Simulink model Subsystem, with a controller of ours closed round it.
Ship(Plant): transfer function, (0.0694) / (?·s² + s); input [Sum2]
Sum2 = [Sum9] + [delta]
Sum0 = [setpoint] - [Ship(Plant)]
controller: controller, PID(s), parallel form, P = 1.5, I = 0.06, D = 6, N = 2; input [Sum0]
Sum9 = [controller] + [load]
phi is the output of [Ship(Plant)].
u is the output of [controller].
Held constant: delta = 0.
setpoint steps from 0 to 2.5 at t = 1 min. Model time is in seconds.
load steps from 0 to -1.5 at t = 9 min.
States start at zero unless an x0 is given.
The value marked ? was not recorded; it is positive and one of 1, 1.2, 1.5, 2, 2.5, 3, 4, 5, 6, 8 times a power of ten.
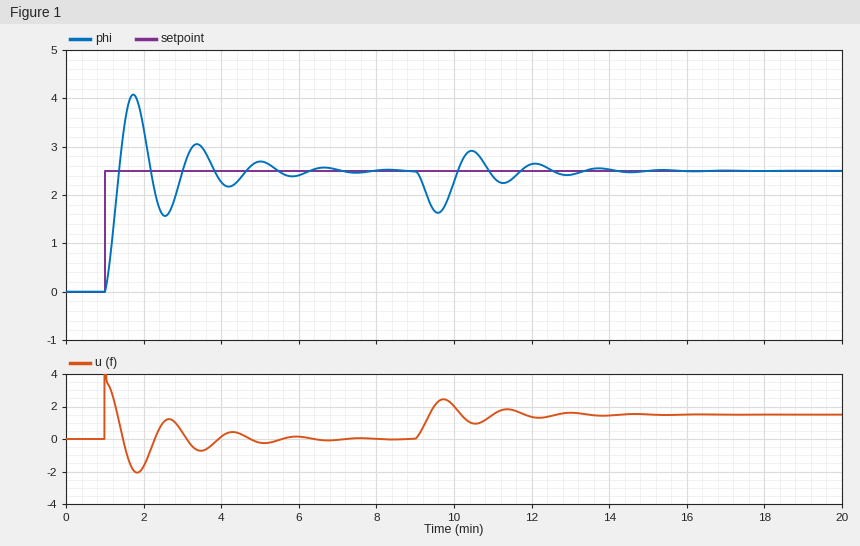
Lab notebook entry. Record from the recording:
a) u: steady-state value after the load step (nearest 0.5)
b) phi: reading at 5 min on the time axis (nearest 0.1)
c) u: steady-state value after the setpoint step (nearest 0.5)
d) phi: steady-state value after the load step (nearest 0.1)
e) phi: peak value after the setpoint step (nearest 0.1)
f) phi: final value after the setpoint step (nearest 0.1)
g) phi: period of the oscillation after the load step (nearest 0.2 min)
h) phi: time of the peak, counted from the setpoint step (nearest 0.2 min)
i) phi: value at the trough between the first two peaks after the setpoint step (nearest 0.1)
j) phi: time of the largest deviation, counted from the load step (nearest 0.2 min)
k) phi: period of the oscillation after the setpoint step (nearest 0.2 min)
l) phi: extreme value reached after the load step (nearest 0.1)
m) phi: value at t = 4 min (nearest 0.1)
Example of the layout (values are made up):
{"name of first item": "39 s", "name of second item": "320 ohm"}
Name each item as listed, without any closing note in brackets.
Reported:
{"u: steady-state value after the load step": "1.5", "phi: reading at 5 min on the time axis": "2.7", "u: steady-state value after the setpoint step": "0.0", "phi: steady-state value after the load step": "2.5", "phi: peak value after the setpoint step": "4.1", "phi: final value after the setpoint step": "2.5", "phi: period of the oscillation after the load step": "1.6 min", "phi: time of the peak, counted from the setpoint step": "0.8 min", "phi: value at the trough between the first two peaks after the setpoint step": "1.6", "phi: time of the largest deviation, counted from the load step": "0.6 min", "phi: period of the oscillation after the setpoint step": "1.6 min", "phi: extreme value reached after the load step": "1.6", "phi: value at t = 4 min": "2.3"}
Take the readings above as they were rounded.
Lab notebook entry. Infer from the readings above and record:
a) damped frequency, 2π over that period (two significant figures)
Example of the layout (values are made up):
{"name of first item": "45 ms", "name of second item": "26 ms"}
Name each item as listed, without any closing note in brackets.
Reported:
{"damped frequency, 2π over that period": "3.9 rad/min"}
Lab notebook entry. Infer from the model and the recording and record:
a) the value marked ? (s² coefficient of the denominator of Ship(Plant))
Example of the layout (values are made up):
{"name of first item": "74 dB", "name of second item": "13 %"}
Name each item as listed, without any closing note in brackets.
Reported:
{"the value marked ? (s² coefficient of the denominator of Ship(Plant))": "20"}
